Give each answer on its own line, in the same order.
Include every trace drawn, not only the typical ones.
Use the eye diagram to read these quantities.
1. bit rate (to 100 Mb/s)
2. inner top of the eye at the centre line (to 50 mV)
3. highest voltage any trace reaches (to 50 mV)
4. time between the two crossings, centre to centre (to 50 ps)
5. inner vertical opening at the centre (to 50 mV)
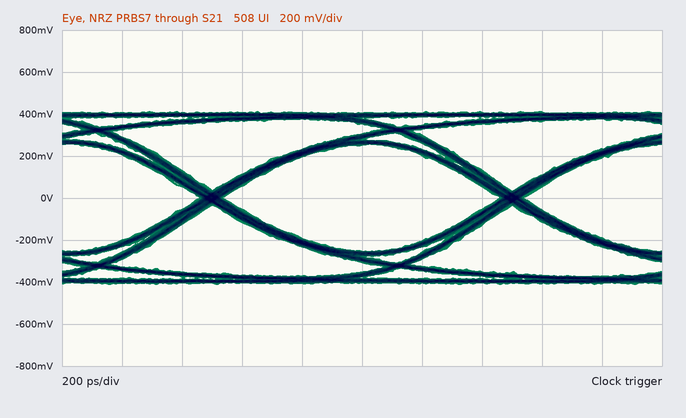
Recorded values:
1.0 Gb/s
250 mV
400 mV
1.00 ns
500 mV
